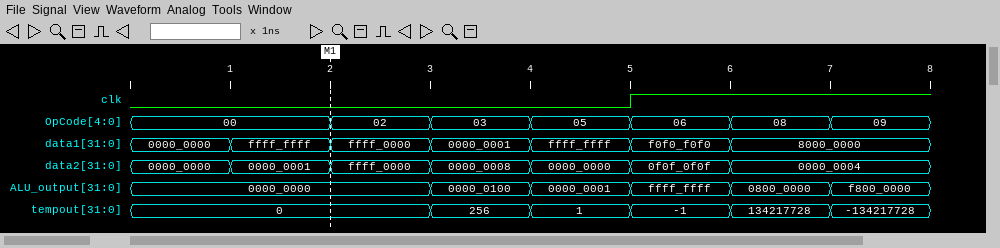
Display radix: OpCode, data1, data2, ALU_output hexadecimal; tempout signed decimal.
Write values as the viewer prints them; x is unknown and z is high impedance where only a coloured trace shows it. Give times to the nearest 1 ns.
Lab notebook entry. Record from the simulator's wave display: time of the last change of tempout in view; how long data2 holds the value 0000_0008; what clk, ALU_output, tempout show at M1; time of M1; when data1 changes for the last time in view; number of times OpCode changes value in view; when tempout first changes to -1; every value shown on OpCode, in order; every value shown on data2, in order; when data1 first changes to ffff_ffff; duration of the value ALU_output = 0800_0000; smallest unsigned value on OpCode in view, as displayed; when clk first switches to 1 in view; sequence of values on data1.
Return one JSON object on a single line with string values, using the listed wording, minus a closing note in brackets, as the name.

{"time of the last change of tempout in view": "7 ns", "how long data2 holds the value 0000_0008": "1 ns", "what clk, ALU_output, tempout show at M1": "clk=0, ALU_output=0000_0000, tempout=0", "time of M1": "2 ns", "when data1 changes for the last time in view": "6 ns", "number of times OpCode changes value in view": "6", "when tempout first changes to -1": "5 ns", "every value shown on OpCode, in order": "00, 02, 03, 05, 06, 08, 09", "every value shown on data2, in order": "0000_0000, 0000_0001, ffff_0000, 0000_0008, 0000_0000, 0f0f_0f0f, 0000_0004", "when data1 first changes to ffff_ffff": "1 ns", "duration of the value ALU_output = 0800_0000": "1 ns", "smallest unsigned value on OpCode in view, as displayed": "00", "when clk first switches to 1 in view": "5 ns", "sequence of values on data1": "0000_0000, ffff_ffff, ffff_0000, 0000_0001, ffff_ffff, f0f0_f0f0, 8000_0000"}
